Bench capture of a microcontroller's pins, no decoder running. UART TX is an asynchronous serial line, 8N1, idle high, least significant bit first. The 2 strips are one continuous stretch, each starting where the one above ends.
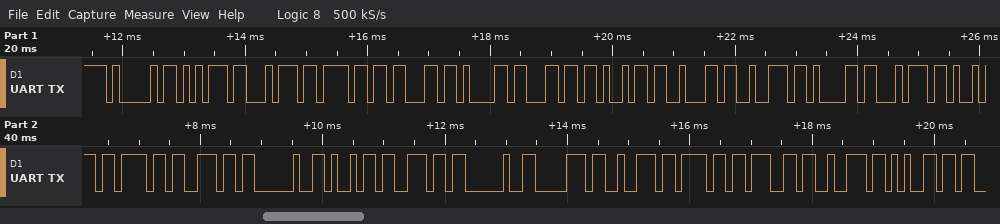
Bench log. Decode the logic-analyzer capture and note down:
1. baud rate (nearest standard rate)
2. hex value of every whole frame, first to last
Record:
9600 baud
41 75 74 6F 63 61 6C 69 62 72 61 74 69 6F 6E 20 69 6E 20 70 72 6F 67 72 65
